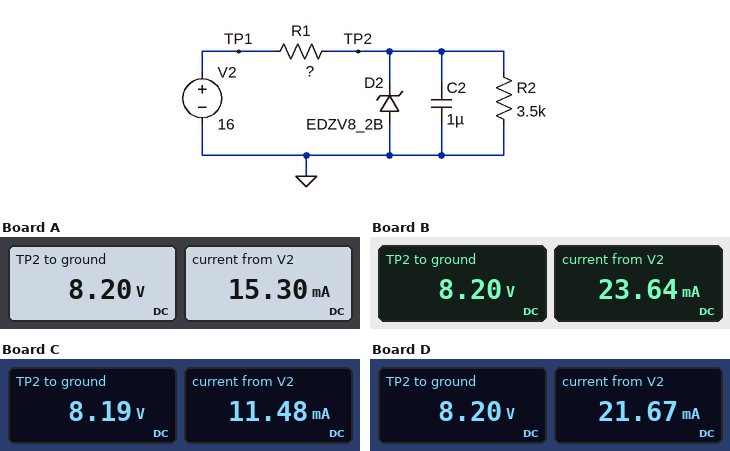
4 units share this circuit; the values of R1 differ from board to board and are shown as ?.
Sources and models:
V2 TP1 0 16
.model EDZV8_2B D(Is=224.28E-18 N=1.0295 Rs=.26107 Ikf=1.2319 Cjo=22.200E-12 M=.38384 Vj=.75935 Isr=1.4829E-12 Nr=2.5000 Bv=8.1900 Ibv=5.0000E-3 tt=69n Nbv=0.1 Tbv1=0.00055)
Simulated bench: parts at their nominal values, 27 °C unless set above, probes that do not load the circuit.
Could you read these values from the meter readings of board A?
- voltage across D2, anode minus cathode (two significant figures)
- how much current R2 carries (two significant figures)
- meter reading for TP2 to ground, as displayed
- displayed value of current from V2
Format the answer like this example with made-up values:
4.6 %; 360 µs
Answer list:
-8.2 V; 2.3 mA; 8.20 V; 15.30 mA
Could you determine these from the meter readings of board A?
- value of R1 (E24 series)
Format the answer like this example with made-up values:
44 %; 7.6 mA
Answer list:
510 Ω
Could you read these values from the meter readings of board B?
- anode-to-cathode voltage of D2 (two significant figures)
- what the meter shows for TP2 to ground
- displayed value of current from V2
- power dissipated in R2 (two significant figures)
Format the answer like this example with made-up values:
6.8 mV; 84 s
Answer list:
-8.2 V; 8.20 V; 23.64 mA; 19 mW
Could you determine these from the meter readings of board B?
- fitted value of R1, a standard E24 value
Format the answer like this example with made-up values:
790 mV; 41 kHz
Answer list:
330 Ω
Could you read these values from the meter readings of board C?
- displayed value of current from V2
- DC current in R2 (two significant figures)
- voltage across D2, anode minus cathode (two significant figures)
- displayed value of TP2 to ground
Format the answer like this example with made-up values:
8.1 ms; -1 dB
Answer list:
11.48 mA; 2.3 mA; -8.2 V; 8.19 V
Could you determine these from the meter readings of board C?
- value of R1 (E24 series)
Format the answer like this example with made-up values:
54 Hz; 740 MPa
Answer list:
680 Ω
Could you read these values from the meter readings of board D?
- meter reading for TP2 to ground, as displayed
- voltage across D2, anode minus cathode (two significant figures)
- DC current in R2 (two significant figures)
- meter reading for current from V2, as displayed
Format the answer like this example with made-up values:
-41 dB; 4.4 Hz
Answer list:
8.20 V; -8.2 V; 2.3 mA; 21.67 mA
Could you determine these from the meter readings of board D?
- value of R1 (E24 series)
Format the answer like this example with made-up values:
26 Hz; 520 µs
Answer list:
360 Ω
